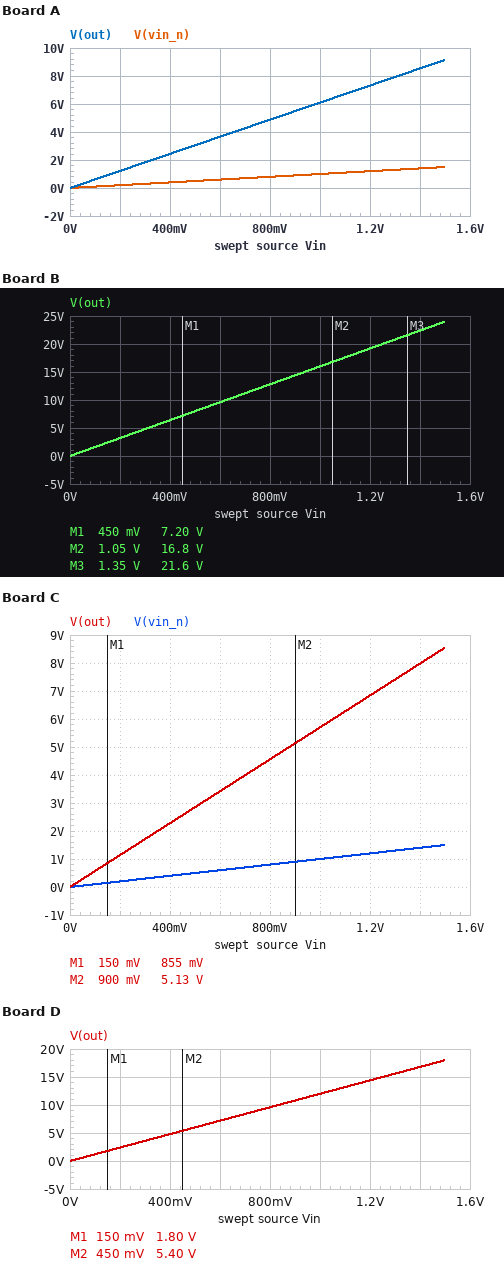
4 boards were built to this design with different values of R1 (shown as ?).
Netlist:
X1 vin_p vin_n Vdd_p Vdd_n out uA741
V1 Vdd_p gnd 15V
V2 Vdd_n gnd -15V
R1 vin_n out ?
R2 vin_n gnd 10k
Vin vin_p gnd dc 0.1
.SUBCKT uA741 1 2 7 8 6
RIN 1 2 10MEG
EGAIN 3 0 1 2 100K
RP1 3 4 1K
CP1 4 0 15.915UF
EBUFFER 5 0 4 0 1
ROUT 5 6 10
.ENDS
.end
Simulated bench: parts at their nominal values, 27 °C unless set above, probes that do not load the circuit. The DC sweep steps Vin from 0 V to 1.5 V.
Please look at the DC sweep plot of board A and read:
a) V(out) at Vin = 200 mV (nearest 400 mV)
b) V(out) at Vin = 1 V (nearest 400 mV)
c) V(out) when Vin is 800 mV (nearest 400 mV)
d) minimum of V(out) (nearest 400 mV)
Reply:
1.2 V
6.0 V
4.8 V
0 V
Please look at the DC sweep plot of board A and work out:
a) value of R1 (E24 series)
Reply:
51 kΩ
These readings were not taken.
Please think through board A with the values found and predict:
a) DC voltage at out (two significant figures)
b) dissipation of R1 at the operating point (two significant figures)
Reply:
610 mV
5.1 µW
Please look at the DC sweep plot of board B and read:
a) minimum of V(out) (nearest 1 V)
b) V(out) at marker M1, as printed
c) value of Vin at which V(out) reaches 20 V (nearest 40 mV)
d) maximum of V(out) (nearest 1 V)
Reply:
0 V
7.20 V
1.24 V
24 V
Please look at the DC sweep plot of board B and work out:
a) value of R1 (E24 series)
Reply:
150 kΩ
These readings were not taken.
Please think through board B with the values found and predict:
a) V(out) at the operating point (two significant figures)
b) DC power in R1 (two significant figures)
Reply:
1.6 V
15 µW
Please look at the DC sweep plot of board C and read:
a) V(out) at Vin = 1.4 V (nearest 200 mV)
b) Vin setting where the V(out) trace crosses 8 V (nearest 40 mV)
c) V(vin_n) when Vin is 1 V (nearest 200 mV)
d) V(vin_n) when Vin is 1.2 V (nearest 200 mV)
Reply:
8.0 V
1.40 V
1.0 V
1.2 V
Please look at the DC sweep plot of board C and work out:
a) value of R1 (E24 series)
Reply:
47 kΩ
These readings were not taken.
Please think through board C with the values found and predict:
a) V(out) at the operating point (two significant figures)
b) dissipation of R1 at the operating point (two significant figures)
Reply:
570 mV
4.7 µW
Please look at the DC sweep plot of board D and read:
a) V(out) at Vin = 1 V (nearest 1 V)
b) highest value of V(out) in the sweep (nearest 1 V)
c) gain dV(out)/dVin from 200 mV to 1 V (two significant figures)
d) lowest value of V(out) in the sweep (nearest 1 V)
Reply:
12 V
18 V
12 V/V
0 V
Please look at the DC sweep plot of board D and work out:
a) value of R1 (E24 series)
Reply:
110 kΩ
